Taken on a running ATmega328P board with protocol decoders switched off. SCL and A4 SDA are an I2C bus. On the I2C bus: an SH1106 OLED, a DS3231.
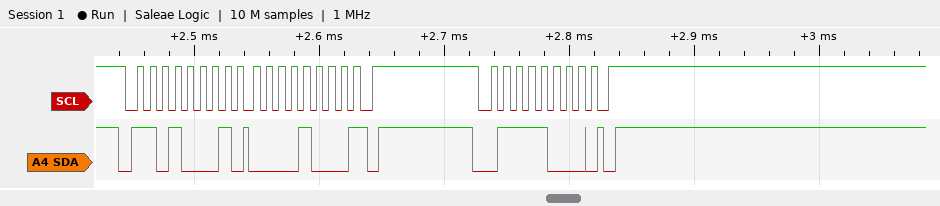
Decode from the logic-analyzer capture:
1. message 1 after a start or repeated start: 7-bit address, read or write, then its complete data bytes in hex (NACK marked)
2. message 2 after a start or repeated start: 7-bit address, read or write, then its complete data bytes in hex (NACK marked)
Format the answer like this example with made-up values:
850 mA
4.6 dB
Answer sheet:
0x68 read: 08 NACK
0x3C write
